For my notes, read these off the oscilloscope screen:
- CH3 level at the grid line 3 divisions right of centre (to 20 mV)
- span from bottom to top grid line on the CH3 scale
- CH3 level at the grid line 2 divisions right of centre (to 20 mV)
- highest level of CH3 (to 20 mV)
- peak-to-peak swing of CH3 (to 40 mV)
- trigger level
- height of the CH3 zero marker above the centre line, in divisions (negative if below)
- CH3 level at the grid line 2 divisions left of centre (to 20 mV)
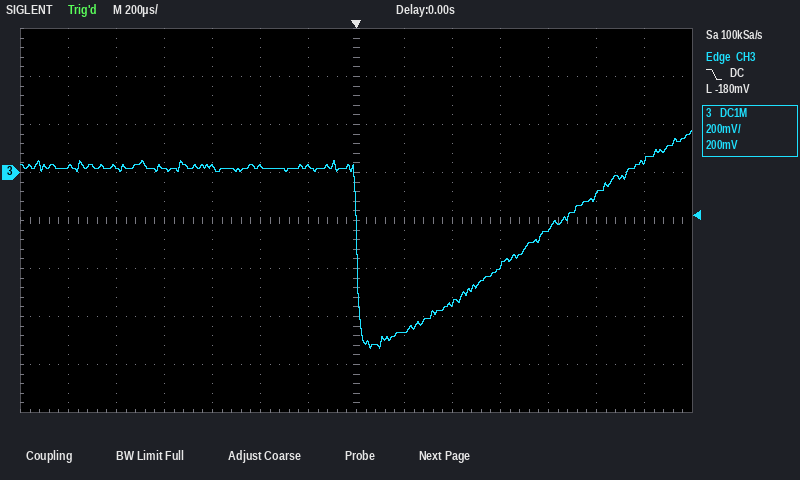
-380 mV
1.6 V
-540 mV
180 mV
920 mV
-180 mV
+1.0 div
20 mV
